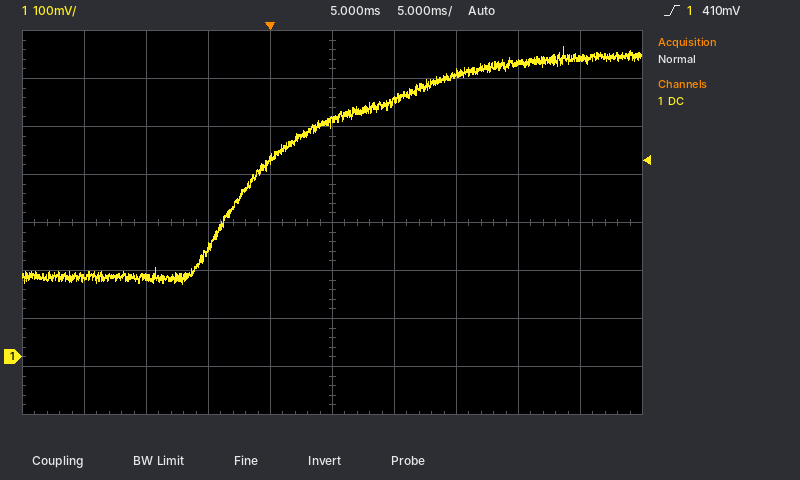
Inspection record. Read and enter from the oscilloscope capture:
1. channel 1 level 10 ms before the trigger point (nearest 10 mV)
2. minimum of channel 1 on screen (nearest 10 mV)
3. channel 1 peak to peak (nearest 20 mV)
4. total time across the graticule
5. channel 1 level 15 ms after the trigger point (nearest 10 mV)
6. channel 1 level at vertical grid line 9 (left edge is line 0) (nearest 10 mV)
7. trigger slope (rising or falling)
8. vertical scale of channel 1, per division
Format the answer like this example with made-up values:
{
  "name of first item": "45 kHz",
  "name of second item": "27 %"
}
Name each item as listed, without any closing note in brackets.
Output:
{
  "channel 1 level 10 ms before the trigger point": "170 mV",
  "minimum of channel 1 on screen": "150 mV",
  "channel 1 peak to peak": "500 mV",
  "total time across the graticule": "50 ms",
  "channel 1 level 15 ms after the trigger point": "590 mV",
  "channel 1 level at vertical grid line 9 (left edge is line 0)": "620 mV",
  "trigger slope": "rising",
  "vertical scale of channel 1, per division": "100 mV"
}
